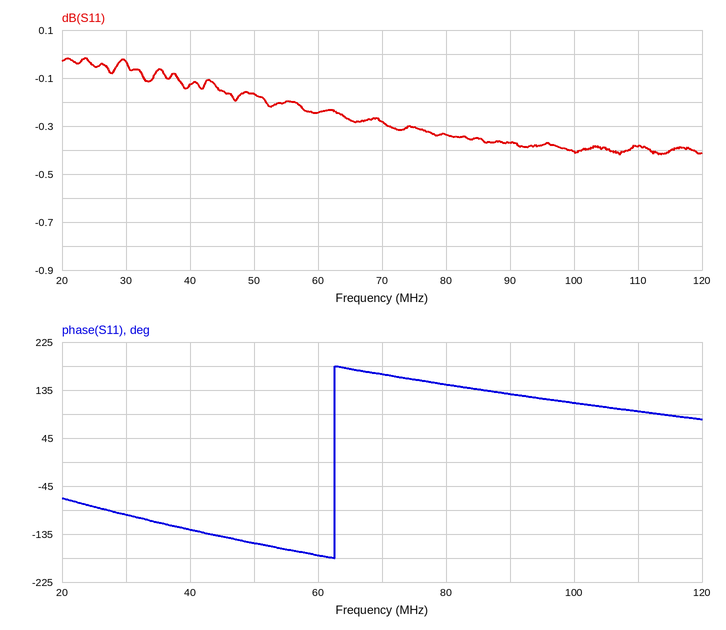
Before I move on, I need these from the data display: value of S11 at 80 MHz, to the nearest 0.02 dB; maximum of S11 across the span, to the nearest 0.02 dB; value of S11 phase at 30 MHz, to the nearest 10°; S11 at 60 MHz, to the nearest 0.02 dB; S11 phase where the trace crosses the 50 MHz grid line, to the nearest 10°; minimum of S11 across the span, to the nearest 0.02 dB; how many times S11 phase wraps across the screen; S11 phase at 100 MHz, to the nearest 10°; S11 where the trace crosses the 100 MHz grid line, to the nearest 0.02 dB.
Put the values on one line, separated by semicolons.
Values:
-0.34 dB; -0.02 dB; -100°; -0.24 dB; -150°; -0.42 dB; 1; 110°; -0.40 dB
